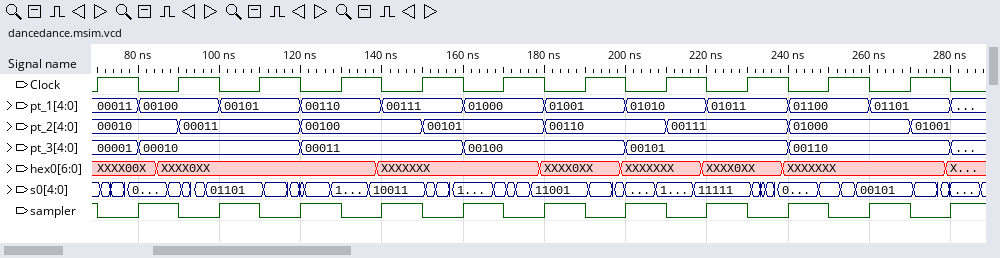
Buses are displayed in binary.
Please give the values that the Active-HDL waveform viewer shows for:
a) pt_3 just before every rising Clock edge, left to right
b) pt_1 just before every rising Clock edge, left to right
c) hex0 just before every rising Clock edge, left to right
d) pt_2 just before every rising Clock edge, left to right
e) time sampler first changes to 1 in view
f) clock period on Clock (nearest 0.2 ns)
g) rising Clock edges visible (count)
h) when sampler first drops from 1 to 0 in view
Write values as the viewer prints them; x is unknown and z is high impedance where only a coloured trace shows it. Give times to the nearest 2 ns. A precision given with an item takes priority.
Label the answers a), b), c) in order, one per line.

a) 00001, 00010, 00010, 00011, 00011, 00100, 00100, 00101, 00101, 00110, 00110
b) 00011, 00100, 00101, 00110, 00111, 01000, 01001, 01010, 01011, 01100, 01101
c) XXXX00X, XXXX0XX, XXXX0XX, XXXX0XX, XXXXXXX, XXXXXXX, XXXX0XX, XXXXXXX, XXXX0XX, XXXXXXX, XXXXXXX
d) 00010, 00010, 00011, 00100, 00100, 00101, 00110, 00110, 00111, 01000, 01000
e) 80 ns
f) 20 ns
g) 11
h) 70 ns
